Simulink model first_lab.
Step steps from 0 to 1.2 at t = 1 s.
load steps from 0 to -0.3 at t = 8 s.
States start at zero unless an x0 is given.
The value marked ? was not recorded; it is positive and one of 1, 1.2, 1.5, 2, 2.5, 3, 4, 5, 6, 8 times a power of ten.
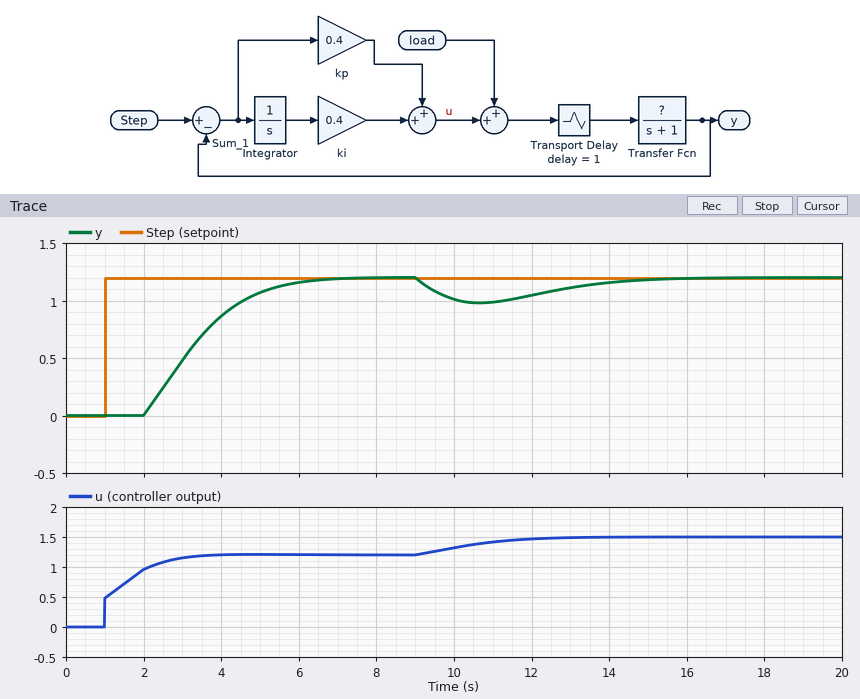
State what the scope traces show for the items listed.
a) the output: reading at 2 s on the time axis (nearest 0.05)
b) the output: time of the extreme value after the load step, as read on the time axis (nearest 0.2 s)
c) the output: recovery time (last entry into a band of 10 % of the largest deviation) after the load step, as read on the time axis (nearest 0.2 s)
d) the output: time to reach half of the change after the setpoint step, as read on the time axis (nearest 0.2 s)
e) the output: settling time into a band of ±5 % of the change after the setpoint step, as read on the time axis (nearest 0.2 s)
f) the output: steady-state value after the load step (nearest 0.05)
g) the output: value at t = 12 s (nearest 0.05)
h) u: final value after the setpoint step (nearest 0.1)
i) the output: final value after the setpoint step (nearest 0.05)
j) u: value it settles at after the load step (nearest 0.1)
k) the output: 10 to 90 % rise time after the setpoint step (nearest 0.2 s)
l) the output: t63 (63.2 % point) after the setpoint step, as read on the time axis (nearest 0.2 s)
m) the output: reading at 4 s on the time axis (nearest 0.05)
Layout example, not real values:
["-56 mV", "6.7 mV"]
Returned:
["0.00", "10.6 s", "14.8 s", "3.2 s", "5.8 s", "1.20", "1.05", "1.2", "1.20", "1.5", "2.8 s", "3.6 s", "0.85"]
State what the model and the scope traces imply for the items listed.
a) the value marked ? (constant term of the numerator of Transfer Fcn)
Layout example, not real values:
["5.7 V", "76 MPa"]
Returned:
["1"]
